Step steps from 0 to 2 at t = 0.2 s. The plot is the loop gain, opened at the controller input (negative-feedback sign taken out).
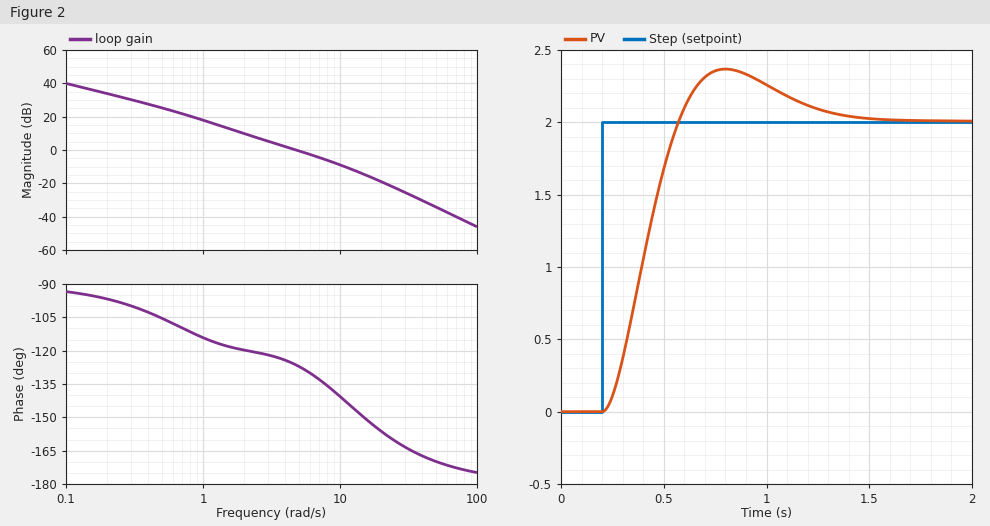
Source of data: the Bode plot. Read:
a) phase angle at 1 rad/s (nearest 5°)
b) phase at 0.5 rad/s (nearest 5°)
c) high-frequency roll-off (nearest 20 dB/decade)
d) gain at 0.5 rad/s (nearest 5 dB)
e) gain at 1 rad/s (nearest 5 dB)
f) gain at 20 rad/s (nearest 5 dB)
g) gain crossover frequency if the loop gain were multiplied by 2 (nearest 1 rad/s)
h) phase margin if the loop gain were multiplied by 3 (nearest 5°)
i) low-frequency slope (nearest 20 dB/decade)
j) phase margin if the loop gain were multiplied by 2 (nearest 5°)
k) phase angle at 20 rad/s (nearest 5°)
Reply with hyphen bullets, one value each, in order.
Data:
- -115°
- -105°
- -40 dB/decade
- 25 dB
- 20 dB
- -20 dB
- 8 rad/s
- 40°
- -20 dB/decade
- 45°
- -155°
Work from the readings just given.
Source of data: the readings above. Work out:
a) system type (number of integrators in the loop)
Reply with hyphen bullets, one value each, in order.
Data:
- 1
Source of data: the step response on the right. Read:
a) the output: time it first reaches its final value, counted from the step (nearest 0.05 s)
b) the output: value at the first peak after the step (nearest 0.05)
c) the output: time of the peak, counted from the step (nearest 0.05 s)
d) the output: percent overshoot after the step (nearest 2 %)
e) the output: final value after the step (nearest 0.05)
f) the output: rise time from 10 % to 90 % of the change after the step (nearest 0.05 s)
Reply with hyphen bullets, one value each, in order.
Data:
- 0.35 s
- 2.35
- 0.60 s
- 18 %
- 2.00
- 0.25 s
